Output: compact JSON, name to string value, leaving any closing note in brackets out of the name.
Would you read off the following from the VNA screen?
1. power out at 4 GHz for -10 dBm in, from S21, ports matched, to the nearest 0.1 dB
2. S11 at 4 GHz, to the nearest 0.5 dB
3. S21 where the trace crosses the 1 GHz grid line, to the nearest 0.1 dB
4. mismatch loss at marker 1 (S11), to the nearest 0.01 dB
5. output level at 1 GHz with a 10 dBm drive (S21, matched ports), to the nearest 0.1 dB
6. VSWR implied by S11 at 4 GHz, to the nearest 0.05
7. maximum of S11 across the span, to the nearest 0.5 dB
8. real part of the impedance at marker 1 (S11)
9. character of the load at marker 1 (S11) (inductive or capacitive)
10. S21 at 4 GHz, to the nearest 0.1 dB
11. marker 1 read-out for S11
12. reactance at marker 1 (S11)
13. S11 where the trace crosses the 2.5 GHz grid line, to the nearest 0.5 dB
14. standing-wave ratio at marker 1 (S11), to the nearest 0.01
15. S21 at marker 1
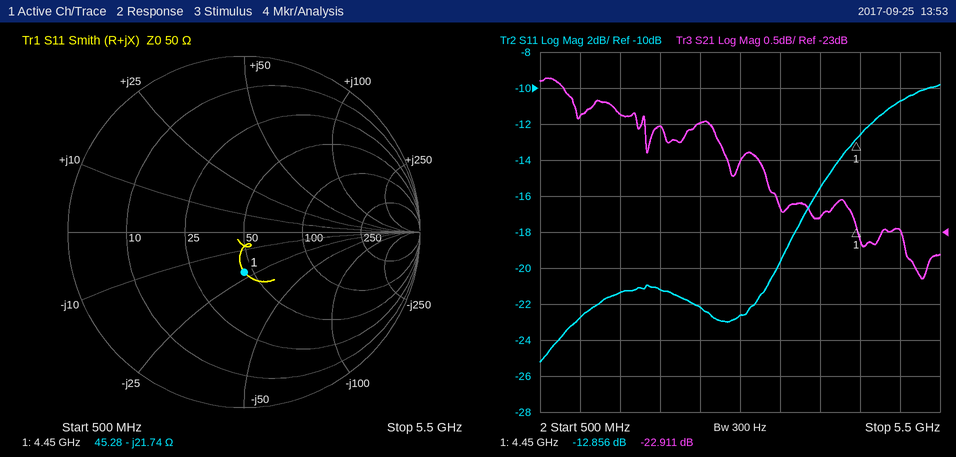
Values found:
{"power out at 4 GHz for -10 dBm in, from S21, ports matched, to the nearest 0.1 dB": "-32.8 dBm", "S11 at 4 GHz, to the nearest 0.5 dB": "-15.5 dB", "S21 where the trace crosses the 1 GHz grid line, to the nearest 0.1 dB": "-21.4 dB", "mismatch loss at marker 1 (S11), to the nearest 0.01 dB": "0.23 dB", "output level at 1 GHz with a 10 dBm drive (S21, matched ports), to the nearest 0.1 dB": "-11.4 dBm", "VSWR implied by S11 at 4 GHz, to the nearest 0.05": "1.40", "maximum of S11 across the span, to the nearest 0.5 dB": "-10.0 dB", "real part of the impedance at marker 1": "45.28 Ω", "character of the load at marker 1 (S11)": "capacitive", "S21 at 4 GHz, to the nearest 0.1 dB": "-22.8 dB", "marker 1 read-out for S11": "-12.856 dB", "reactance at marker 1": "-21.74 Ω", "S11 where the trace crosses the 2.5 GHz grid line, to the nearest 0.5 dB": "-22.0 dB", "standing-wave ratio at marker 1 (S11), to the nearest 0.01": "1.59", "S21 at marker 1": "-22.911 dB"}
